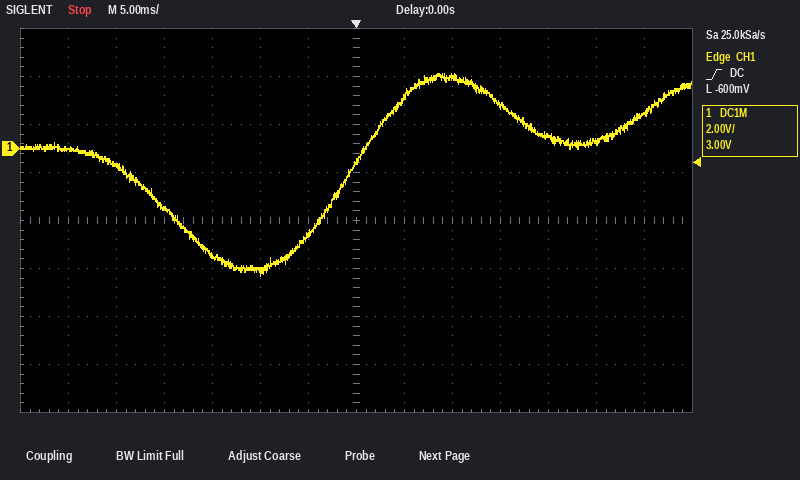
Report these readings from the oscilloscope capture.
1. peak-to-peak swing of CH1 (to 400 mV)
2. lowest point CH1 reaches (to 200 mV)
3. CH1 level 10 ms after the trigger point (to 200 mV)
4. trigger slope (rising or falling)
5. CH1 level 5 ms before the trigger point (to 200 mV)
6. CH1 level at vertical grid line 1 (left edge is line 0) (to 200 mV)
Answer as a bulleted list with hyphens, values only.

- 8.4 V
- -5.2 V
- 3.0 V
- rising
- -3.6 V
- 0.0 V
